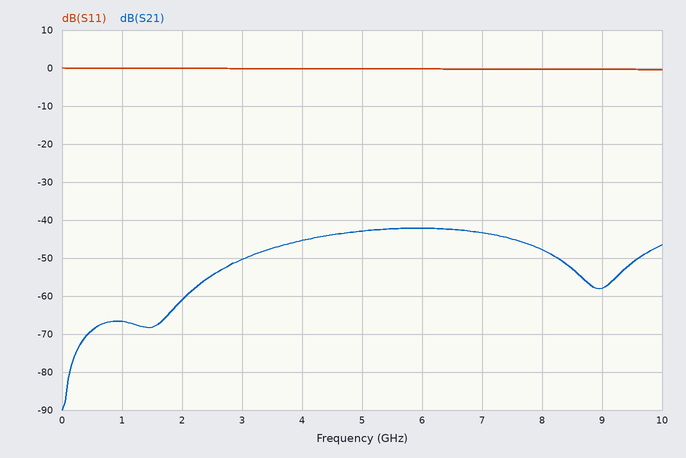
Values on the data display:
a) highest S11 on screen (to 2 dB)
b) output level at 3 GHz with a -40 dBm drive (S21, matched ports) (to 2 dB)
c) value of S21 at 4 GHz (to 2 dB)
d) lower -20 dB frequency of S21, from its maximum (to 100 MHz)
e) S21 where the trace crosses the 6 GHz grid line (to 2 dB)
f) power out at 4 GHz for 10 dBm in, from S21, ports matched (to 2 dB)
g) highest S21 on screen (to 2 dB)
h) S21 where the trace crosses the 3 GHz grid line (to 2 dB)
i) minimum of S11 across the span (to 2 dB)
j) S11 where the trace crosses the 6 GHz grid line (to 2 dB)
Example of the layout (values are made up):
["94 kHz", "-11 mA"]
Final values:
["0 dB", "-90 dBm", "-46 dB", "1.9 GHz", "-42 dB", "-36 dBm", "-42 dB", "-50 dB", "0 dB", "0 dB"]
